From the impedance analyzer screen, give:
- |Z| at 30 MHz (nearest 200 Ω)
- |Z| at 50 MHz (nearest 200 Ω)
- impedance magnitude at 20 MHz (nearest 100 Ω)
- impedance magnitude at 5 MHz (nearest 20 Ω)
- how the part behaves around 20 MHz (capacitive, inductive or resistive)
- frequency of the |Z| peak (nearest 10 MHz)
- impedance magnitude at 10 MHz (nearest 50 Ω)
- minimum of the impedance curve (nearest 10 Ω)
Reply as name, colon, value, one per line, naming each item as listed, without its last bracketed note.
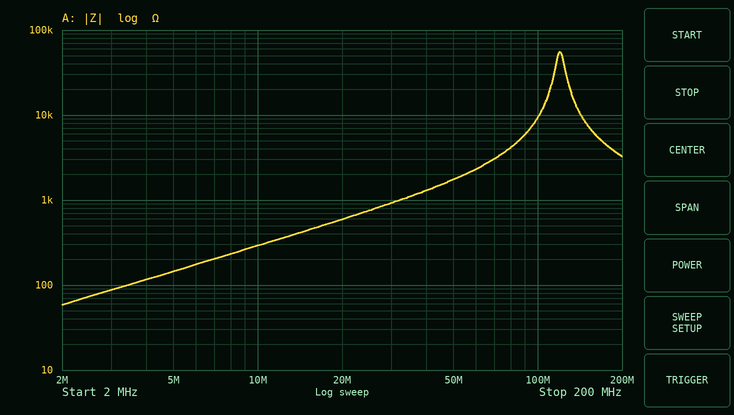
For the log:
|Z| at 30 MHz: 1.0 kΩ
|Z| at 50 MHz: 1.8 kΩ
impedance magnitude at 20 MHz: 600 Ω
impedance magnitude at 5 MHz: 140 Ω
how the part behaves around 20 MHz: inductive
frequency of the |Z| peak: 120 MHz
impedance magnitude at 10 MHz: 300 Ω
minimum of the impedance curve: 60 Ω
